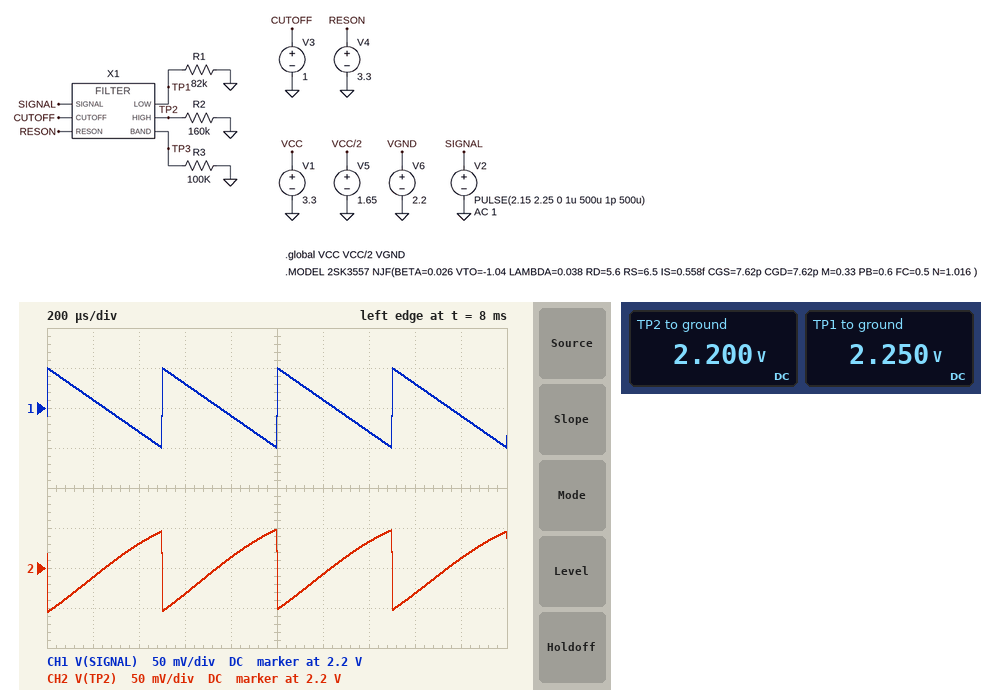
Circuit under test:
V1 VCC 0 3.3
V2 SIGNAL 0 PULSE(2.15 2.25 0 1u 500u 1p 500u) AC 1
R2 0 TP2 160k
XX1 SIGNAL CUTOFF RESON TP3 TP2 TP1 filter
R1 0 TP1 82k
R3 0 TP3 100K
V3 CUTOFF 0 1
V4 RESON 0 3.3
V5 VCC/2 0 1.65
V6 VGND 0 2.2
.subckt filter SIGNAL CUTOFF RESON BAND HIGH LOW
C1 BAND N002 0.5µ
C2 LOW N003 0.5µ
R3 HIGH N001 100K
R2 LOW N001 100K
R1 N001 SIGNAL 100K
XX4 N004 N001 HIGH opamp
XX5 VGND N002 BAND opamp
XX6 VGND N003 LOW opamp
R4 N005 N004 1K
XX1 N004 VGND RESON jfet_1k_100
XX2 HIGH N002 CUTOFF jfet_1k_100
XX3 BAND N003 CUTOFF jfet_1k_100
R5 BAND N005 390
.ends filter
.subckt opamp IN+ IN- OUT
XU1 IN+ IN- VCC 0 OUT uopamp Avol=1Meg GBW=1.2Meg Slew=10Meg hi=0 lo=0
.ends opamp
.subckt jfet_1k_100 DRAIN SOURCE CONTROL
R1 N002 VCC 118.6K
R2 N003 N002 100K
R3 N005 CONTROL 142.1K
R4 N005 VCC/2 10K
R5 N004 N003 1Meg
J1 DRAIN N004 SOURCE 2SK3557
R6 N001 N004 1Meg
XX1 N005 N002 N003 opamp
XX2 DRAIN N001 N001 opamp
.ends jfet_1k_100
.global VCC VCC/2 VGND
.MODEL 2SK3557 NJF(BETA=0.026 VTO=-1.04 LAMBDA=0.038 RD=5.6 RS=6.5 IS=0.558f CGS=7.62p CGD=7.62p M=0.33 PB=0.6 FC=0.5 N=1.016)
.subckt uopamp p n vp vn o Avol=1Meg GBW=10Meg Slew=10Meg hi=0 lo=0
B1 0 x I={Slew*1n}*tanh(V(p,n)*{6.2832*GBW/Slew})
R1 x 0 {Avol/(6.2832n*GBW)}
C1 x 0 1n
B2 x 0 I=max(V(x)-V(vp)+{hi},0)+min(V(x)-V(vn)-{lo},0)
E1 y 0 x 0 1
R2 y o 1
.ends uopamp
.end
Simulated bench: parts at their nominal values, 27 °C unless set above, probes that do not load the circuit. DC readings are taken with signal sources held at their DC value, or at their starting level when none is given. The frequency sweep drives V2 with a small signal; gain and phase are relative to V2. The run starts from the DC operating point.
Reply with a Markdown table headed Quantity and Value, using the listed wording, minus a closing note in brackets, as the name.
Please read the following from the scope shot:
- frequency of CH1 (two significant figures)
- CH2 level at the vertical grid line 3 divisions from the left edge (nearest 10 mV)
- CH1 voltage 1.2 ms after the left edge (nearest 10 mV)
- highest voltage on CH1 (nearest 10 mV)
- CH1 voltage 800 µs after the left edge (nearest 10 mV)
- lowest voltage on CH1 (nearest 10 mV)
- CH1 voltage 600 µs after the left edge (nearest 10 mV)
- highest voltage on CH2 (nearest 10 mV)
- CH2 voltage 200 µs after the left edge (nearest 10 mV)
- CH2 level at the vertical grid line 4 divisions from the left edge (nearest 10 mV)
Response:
| Quantity | Value |
|---|---|
| frequency of CH1 | 2.0 kHz |
| CH2 level at the vertical grid line 3 divisions from the left edge | 2.17 V |
| CH1 voltage 1.2 ms after the left edge | 2.21 V |
| highest voltage on CH1 | 2.25 V |
| CH1 voltage 800 µs after the left edge | 2.19 V |
| lowest voltage on CH1 | 2.15 V |
| CH1 voltage 600 µs after the left edge | 2.23 V |
| highest voltage on CH2 | 2.25 V |
| CH2 voltage 200 µs after the left edge | 2.19 V |
| CH2 level at the vertical grid line 4 divisions from the left edge | 2.21 V |
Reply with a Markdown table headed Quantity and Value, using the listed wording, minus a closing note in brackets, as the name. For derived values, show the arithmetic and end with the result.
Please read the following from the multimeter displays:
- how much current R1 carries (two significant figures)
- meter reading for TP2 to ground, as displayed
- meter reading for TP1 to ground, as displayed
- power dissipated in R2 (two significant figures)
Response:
| Quantity | Value |
|---|---|
| how much current R1 carries | (2.25 V) / 82 kΩ = 27 µA |
| meter reading for TP2 to ground, as displayed | 2.200 V |
| meter reading for TP1 to ground, as displayed | 2.250 V |
| power dissipated in R2 | (2.2 V)^2 / 160 kΩ = 30 µW |
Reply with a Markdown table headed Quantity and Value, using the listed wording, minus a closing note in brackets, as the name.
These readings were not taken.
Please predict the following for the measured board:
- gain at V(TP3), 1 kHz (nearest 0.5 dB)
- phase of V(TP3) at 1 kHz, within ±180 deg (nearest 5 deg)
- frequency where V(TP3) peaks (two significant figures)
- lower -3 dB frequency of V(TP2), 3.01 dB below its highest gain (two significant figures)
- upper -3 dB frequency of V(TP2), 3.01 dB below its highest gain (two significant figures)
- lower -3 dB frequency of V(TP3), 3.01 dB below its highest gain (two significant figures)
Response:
| Quantity | Value |
|---|---|
| gain at V(TP3), 1 kHz | -4.0 dB |
| phase of V(TP3) at 1 kHz, within ±180 deg | -80 deg |
| frequency where V(TP3) peaks | 490 Hz |
| lower -3 dB frequency of V(TP2), 3.01 dB below its highest gain | 440 Hz |
| upper -3 dB frequency of V(TP2), 3.01 dB below its highest gain | 570 Hz |
| lower -3 dB frequency of V(TP3), 3.01 dB below its highest gain | 430 Hz |
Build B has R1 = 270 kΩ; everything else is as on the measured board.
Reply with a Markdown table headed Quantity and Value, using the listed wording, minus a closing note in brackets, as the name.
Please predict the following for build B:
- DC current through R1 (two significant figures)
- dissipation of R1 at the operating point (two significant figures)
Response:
| Quantity | Value |
|---|---|
| DC current through R1 | 8.3 µA |
| dissipation of R1 at the operating point | 19 µW |
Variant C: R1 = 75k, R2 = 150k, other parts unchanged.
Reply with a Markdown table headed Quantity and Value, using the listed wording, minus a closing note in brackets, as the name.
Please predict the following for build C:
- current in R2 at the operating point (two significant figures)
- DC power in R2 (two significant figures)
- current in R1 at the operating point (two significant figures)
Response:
| Quantity | Value |
|---|---|
| current in R2 at the operating point | 15 µA |
| DC power in R2 | 32 µW |
| current in R1 at the operating point | 30 µA |
